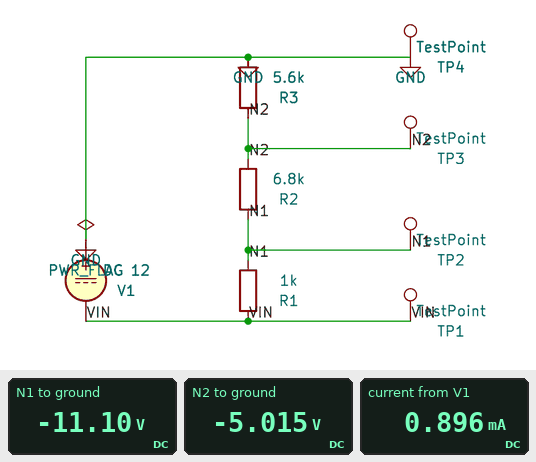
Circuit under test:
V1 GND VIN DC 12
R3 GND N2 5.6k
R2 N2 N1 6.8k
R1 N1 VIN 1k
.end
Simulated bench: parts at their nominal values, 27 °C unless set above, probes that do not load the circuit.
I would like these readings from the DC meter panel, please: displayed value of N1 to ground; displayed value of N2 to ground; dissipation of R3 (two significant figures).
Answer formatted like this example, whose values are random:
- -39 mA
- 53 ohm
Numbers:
- -11.10 V
- -5.015 V
- 4.5 mW
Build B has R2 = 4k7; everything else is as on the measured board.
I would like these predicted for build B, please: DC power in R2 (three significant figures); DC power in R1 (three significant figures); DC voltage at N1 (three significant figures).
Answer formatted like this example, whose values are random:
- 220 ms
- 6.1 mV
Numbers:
- 5.30 mW
- 1.13 mW
- -10.9 V
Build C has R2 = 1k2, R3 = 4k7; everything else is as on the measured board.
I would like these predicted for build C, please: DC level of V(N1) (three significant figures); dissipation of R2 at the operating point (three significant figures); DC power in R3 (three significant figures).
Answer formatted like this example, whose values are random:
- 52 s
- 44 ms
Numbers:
- -10.3 V
- 3.63 mW
- 14.2 mW
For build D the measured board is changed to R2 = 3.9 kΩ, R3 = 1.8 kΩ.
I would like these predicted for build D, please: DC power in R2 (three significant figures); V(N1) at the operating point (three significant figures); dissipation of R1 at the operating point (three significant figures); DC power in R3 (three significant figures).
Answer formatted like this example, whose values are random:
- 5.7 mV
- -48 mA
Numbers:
- 12.5 mW
- -10.2 V
- 3.21 mW
- 5.77 mW
